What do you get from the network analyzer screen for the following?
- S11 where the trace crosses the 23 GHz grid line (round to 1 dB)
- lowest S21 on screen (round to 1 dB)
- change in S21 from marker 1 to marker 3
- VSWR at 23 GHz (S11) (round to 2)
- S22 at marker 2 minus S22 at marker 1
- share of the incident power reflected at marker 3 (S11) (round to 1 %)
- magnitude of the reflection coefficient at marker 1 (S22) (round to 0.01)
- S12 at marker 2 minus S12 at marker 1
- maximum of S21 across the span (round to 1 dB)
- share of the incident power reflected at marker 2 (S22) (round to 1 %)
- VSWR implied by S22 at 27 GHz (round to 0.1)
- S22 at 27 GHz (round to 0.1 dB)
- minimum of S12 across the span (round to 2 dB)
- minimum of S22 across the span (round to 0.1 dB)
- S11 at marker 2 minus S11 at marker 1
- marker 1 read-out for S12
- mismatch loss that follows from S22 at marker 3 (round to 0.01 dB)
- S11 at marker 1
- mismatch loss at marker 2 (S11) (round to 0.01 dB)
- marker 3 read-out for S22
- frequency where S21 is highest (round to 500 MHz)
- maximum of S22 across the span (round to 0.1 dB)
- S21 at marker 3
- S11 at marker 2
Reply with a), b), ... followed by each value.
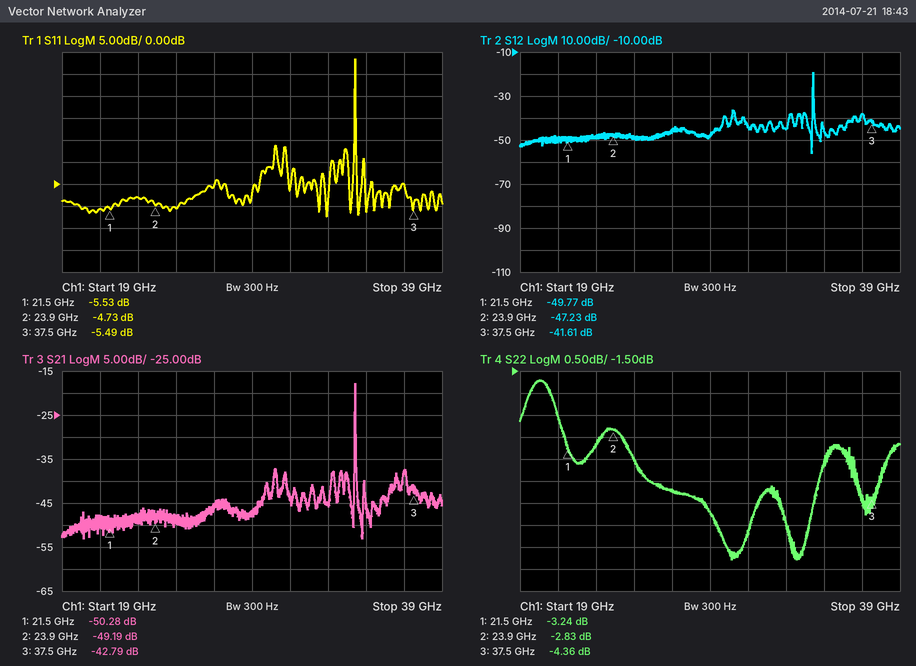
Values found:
a) -3 dB
b) -53 dB
c) 7.49 dB
d) 6
e) 0.41 dB
f) 28 %
g) 0.69
h) 2.54 dB
i) -18 dB
j) 52 %
k) 4.2
l) -4.2 dB
m) -56 dB
n) -5.8 dB
o) 0.80 dB
p) -49.77 dB
q) 1.98 dB
r) -5.53 dB
s) 1.78 dB
t) -4.36 dB
u) 34.5 GHz
v) -1.7 dB
w) -42.79 dB
x) -4.73 dB
